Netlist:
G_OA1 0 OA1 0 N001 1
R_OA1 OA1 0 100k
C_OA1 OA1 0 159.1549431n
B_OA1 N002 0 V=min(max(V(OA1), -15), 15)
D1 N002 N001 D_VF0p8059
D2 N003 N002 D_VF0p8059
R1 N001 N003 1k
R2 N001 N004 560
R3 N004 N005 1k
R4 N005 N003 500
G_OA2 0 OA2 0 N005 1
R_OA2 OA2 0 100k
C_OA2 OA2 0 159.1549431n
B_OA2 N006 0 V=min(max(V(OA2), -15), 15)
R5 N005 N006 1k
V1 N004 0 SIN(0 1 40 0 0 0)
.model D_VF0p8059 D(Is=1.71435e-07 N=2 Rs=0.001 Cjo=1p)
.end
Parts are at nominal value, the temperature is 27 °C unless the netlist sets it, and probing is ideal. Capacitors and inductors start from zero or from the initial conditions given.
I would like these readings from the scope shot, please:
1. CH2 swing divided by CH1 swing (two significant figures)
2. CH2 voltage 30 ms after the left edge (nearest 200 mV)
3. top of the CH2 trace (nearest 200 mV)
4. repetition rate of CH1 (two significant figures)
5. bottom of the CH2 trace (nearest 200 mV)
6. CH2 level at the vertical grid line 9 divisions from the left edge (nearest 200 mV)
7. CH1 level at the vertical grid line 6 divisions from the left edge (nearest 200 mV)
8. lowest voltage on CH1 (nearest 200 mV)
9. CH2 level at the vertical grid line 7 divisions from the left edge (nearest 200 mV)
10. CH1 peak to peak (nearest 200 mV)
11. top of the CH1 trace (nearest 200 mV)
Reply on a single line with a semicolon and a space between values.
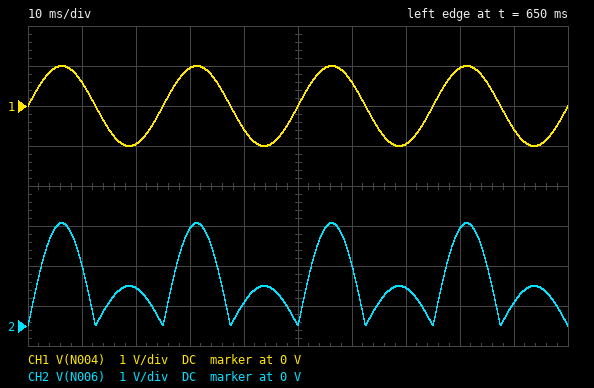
1.3; 2.4 V; 2.6 V; 40 Hz; 0 V; 600 mV; 600 mV; -1.0 V; 1.0 V; 2.0 V; 1.0 V
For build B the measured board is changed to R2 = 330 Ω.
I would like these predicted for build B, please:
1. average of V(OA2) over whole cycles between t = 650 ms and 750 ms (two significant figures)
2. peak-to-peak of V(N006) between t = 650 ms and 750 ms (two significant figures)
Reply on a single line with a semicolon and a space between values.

1.9 V; 5.1 V
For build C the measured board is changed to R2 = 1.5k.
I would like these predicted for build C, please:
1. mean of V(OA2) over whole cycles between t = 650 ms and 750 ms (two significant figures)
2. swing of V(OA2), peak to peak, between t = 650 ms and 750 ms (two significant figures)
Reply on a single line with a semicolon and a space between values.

420 mV; 1.0 V
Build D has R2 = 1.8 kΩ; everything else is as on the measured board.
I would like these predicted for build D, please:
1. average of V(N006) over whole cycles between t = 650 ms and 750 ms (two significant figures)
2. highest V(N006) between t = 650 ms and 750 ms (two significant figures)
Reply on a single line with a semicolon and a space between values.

350 mV; 1.0 V
